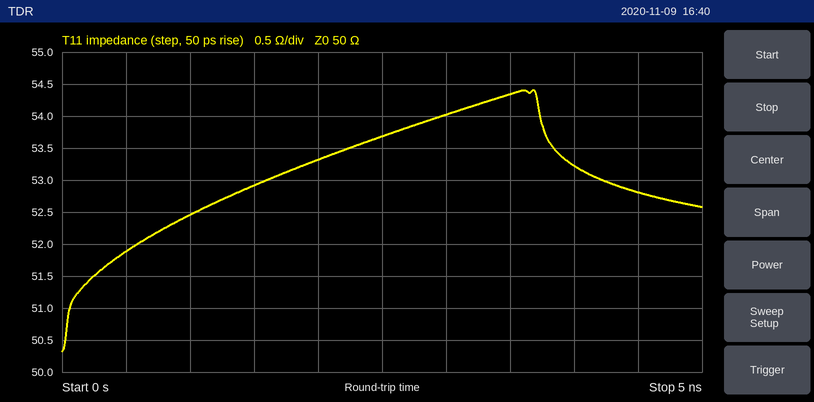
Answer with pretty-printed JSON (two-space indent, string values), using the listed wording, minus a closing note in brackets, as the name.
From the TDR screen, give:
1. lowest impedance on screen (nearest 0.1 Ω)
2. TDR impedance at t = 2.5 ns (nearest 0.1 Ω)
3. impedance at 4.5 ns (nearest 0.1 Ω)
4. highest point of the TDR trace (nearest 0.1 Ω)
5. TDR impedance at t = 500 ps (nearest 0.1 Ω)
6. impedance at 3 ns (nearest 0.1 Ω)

{
  "lowest impedance on screen": "50.3 Ω",
  "TDR impedance at t = 2.5 ns": "53.7 Ω",
  "impedance at 4.5 ns": "52.8 Ω",
  "highest point of the TDR trace": "54.4 Ω",
  "TDR impedance at t = 500 ps": "51.9 Ω",
  "impedance at 3 ns": "54.0 Ω"
}
